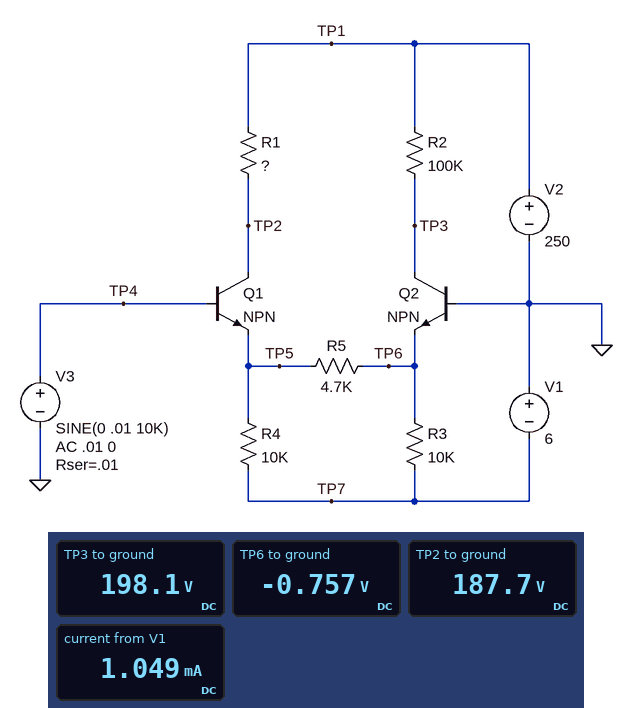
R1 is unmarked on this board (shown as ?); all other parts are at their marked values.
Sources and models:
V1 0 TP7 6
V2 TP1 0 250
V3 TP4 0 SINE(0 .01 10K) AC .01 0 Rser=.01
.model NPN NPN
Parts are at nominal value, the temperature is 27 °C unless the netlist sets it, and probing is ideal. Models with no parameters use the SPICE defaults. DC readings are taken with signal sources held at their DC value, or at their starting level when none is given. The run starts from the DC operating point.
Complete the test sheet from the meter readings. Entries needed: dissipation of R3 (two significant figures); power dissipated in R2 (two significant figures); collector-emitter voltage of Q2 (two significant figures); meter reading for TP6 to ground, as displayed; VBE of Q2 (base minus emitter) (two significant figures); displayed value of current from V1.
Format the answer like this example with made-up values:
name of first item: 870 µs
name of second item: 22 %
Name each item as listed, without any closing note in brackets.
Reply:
dissipation of R3: 2.7 mW
power dissipated in R2: 27 mW
collector-emitter voltage of Q2: 200 V
meter reading for TP6 to ground, as displayed: -0.757 V
VBE of Q2 (base minus emitter): 760 mV
displayed value of current from V1: 1.049 mA
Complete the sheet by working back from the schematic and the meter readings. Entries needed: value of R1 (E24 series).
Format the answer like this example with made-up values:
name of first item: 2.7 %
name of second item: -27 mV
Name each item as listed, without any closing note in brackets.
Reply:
value of R1: 120 kΩ
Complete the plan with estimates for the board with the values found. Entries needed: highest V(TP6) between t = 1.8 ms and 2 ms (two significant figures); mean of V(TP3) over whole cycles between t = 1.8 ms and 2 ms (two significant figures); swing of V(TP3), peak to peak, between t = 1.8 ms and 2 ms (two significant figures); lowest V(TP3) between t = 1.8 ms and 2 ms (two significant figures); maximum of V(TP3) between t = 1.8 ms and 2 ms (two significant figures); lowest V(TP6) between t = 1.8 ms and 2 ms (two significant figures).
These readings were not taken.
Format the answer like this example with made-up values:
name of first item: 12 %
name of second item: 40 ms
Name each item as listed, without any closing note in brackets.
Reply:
highest V(TP6) between t = 1.8 ms and 2 ms: -760 mV
mean of V(TP3) over whole cycles between t = 1.8 ms and 2 ms: 200 V
swing of V(TP3), peak to peak, between t = 1.8 ms and 2 ms: 410 mV
lowest V(TP3) between t = 1.8 ms and 2 ms: 200 V
maximum of V(TP3) between t = 1.8 ms and 2 ms: 200 V
lowest V(TP6) between t = 1.8 ms and 2 ms: -760 mV
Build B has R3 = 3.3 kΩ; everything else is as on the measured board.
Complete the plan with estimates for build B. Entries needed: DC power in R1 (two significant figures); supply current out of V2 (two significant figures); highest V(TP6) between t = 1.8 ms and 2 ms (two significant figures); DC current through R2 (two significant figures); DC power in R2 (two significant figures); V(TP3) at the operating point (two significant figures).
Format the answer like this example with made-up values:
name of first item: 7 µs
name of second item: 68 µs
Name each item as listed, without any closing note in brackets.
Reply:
DC power in R1: 33 mW
supply current out of V2: 2.1 mA
highest V(TP6) between t = 1.8 ms and 2 ms: -790 mV
DC current through R2: 1.6 mA
DC power in R2: 240 mW
V(TP3) at the operating point: 94 V
